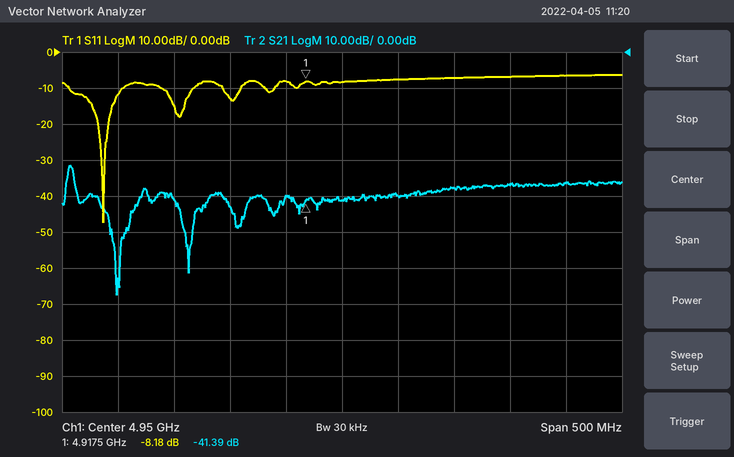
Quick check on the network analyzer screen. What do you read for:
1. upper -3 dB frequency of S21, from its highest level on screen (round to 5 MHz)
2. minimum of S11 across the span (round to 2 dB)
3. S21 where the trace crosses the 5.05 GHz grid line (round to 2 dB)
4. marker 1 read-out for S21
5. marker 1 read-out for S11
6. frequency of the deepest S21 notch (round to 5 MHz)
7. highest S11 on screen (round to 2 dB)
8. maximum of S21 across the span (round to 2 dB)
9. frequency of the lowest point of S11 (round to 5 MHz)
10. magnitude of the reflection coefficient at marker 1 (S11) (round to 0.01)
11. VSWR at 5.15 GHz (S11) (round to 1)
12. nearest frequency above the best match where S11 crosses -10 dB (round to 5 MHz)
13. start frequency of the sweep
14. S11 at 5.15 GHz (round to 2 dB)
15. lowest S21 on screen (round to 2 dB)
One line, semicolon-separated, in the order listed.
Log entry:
4.710 GHz; -48 dB; -38 dB; -41.39 dB; -8.18 dB; 4.750 GHz; -6 dB; -32 dB; 4.735 GHz; 0.39; 3; 4.755 GHz; 4.7 GHz; -6 dB; -68 dB
